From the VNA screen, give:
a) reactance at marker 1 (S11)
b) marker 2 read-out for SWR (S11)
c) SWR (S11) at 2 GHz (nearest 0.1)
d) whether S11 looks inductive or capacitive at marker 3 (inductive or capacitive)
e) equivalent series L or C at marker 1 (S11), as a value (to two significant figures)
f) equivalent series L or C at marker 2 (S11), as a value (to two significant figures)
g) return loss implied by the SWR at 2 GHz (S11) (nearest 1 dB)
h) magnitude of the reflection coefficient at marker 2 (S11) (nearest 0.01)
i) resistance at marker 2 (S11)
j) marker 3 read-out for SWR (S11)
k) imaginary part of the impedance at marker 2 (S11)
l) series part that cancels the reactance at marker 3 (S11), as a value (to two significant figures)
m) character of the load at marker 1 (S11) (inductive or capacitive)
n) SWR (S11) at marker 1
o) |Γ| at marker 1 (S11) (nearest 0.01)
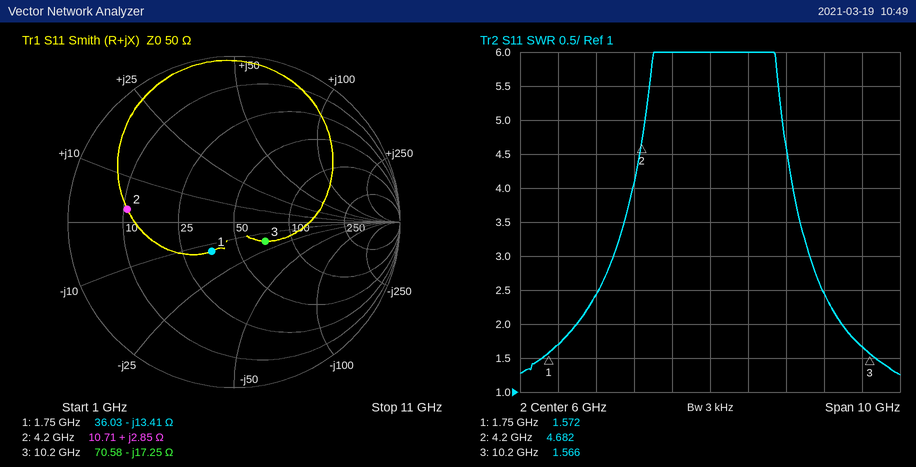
-13.41 Ω
4.682
1.7
capacitive
6.8 pF
110 pH
12 dB
0.65
10.71 Ω
1.566
+2.85 Ω
270 pH
capacitive
1.572
0.22
